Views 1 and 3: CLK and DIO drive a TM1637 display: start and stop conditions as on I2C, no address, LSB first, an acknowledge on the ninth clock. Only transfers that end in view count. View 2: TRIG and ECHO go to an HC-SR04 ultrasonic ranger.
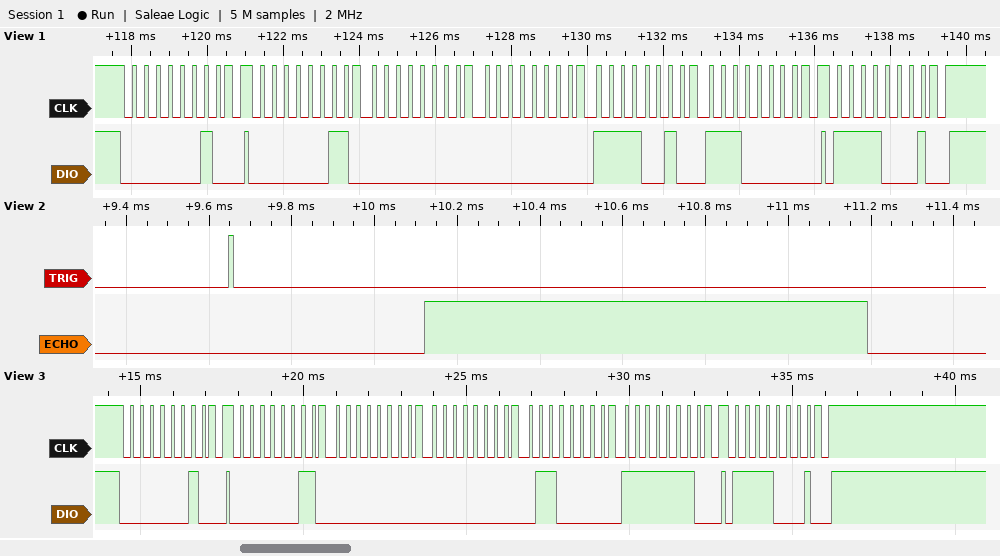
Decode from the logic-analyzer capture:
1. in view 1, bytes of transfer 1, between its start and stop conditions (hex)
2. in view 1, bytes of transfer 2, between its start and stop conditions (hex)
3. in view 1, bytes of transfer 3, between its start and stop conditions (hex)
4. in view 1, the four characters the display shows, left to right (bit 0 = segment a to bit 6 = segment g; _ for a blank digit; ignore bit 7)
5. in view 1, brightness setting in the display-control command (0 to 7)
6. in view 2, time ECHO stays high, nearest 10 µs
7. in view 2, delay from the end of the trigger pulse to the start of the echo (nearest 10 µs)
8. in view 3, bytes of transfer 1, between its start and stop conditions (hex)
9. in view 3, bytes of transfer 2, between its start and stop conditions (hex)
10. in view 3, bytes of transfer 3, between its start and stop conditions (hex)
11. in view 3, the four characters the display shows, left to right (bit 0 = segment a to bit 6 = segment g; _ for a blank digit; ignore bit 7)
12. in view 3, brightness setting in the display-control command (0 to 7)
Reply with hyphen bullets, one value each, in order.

- 40
- C0 00 00 4F 07
- 8F
- __37
- 7
- 1070 µs
- 460 µs
- 40
- C0 00 00 06 7F
- 8F
- __18
- 7
